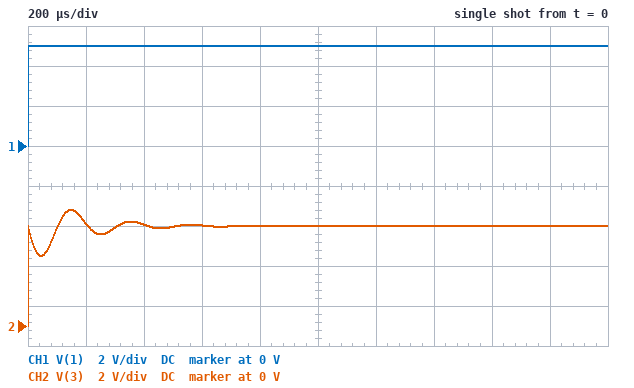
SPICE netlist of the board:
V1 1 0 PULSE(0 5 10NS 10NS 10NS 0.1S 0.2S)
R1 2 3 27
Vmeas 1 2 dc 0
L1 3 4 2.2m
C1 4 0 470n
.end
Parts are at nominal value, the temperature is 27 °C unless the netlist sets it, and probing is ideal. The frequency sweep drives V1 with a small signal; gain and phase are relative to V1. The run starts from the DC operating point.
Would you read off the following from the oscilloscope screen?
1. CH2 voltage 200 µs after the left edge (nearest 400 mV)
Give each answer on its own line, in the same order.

5.2 V
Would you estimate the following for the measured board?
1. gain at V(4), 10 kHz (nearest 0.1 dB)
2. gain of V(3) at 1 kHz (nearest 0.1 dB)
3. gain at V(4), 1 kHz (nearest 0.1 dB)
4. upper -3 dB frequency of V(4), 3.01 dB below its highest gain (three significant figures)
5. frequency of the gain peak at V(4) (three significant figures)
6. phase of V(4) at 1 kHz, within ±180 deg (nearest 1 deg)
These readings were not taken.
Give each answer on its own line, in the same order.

-10.1 dB
0 dB
0.3 dB
5.66 kHz
4.75 kHz
-5 deg
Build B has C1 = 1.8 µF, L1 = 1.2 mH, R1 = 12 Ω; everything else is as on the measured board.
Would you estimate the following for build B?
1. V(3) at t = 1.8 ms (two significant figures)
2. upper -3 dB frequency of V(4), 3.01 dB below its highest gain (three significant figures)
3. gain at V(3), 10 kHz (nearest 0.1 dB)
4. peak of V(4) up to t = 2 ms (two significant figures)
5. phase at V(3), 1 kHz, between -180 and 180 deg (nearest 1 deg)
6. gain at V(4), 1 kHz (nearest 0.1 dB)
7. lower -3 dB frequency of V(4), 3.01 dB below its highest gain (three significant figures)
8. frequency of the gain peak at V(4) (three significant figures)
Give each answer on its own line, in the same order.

5.0 V
3.97 kHz
-0.1 dB
7.4 V
-8 deg
0.7 dB
2.27 kHz
3.23 kHz
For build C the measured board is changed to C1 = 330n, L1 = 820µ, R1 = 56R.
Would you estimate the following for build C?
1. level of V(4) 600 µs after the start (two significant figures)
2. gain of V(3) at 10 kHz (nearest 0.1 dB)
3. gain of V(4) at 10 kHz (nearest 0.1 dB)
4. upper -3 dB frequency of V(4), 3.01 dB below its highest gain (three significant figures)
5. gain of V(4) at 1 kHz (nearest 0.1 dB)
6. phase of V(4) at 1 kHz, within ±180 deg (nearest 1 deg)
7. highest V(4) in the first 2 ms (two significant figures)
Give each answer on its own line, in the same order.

5.0 V
-24.6 dB
-1.3 dB
11.0 kHz
0 dB
-7 deg
5.6 V
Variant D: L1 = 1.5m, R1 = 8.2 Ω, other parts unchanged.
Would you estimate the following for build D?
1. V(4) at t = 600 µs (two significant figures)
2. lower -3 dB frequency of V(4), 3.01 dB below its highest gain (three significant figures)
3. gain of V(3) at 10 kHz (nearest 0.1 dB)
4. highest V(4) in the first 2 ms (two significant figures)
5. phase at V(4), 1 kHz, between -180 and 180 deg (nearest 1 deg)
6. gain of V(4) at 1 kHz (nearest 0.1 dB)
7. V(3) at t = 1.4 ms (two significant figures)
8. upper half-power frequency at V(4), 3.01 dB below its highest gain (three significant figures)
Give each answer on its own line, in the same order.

5.9 V
5.51 kHz
-0.1 dB
9.0 V
-1 deg
0.2 dB
5.0 V
6.38 kHz
